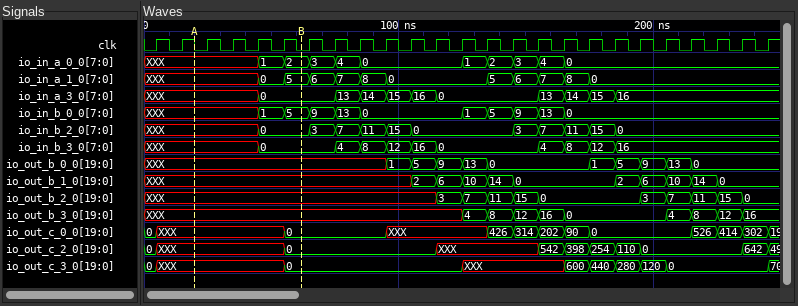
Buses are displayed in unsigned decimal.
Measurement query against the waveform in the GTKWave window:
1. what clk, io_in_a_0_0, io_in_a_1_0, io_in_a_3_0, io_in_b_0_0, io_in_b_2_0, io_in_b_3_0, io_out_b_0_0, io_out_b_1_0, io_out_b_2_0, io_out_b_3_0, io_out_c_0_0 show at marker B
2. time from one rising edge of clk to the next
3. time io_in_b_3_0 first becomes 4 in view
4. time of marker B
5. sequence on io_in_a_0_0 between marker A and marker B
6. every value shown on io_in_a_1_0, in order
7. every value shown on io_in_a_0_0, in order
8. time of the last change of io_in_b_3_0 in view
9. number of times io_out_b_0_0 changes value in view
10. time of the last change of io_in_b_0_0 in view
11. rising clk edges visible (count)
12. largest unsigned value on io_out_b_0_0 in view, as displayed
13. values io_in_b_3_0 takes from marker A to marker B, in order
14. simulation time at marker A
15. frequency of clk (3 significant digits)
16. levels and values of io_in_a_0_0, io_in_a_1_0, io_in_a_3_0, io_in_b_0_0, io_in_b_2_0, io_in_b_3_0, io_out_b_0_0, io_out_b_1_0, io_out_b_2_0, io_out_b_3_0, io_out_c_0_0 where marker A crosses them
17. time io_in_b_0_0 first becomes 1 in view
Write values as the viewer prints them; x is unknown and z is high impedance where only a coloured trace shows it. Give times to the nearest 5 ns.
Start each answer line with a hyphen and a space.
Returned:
- clk=0, io_in_a_0_0=2, io_in_a_1_0=5, io_in_a_3_0=0, io_in_b_0_0=5, io_in_b_2_0=0, io_in_b_3_0=0, io_out_b_0_0=XXX, io_out_b_1_0=XXX, io_out_b_2_0=XXX, io_out_b_3_0=XXX, io_out_c_0_0=0
- 10 ns
- 75 ns
- 60 ns
- XXX, 1, 2
- XXX, 0, 5, 6, 7, 8, 0, 5, 6, 7, 8, 0
- XXX, 1, 2, 3, 4, 0, 1, 2, 3, 4, 0
- 185 ns
- 10
- 165 ns
- 25
- 13
- XXX, 0
- 20 ns
- 100 MHz
- io_in_a_0_0=XXX, io_in_a_1_0=XXX, io_in_a_3_0=XXX, io_in_b_0_0=XXX, io_in_b_2_0=XXX, io_in_b_3_0=XXX, io_out_b_0_0=XXX, io_out_b_1_0=XXX, io_out_b_2_0=XXX, io_out_b_3_0=XXX, io_out_c_0_0=XXX
- 45 ns
